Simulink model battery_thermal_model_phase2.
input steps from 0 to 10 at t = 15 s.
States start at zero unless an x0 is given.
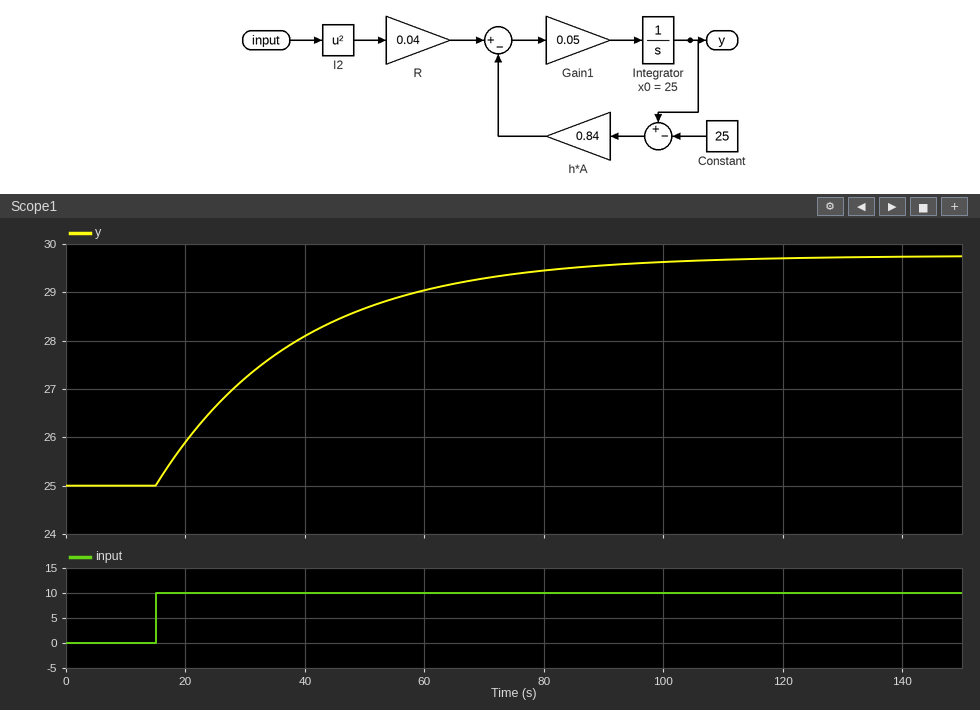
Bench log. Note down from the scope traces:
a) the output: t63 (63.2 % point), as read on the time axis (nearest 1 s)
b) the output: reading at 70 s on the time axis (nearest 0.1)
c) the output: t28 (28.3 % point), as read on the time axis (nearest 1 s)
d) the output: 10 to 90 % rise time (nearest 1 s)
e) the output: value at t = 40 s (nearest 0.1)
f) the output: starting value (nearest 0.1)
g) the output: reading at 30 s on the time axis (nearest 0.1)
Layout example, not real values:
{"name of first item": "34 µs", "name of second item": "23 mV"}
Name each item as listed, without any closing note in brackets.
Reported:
{"the output: t63 (63.2 % point), as read on the time axis": "39 s", "the output: reading at 70 s on the time axis": "29.3", "the output: t28 (28.3 % point), as read on the time axis": "23 s", "the output: 10 to 90 % rise time": "52 s", "the output: value at t = 40 s": "28.1", "the output: starting value": "25.0", "the output: reading at 30 s on the time axis": "27.2"}
